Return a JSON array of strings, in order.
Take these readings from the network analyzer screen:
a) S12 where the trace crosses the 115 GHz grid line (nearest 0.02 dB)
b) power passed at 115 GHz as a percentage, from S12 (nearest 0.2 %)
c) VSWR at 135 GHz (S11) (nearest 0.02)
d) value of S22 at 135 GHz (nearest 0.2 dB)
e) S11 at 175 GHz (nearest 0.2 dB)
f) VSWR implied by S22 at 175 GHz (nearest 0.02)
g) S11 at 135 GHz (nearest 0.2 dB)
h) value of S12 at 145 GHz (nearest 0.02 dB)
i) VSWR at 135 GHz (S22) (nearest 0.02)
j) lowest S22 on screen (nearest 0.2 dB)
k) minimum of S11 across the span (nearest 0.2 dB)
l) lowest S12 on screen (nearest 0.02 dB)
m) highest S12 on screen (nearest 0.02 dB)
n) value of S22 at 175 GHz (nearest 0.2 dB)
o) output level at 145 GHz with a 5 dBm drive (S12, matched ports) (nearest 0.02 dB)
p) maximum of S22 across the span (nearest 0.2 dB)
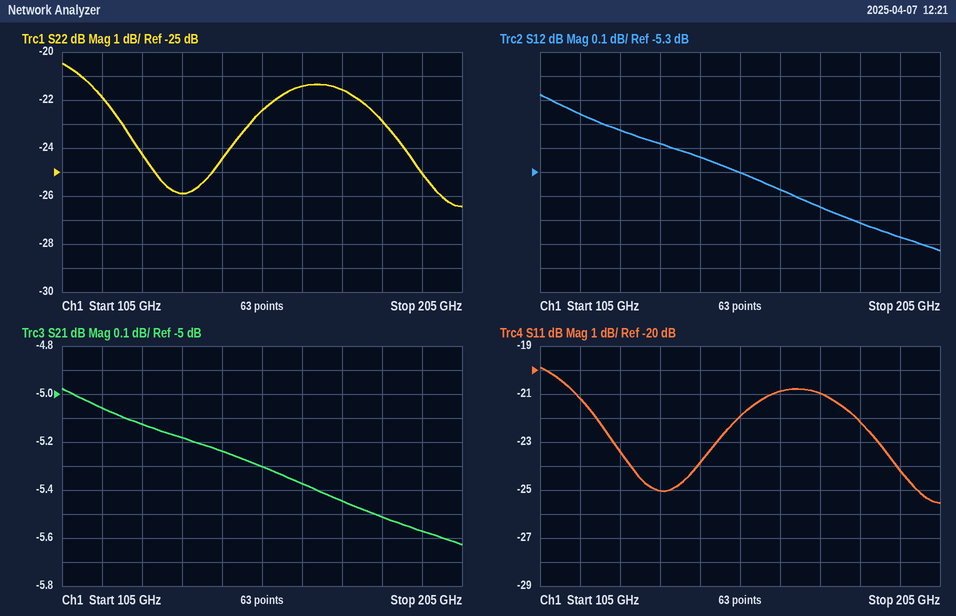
["-5.06 dB", "31.2 %", "1.12", "-25.8 dB", "-21.0 dB", "1.18", "-25.0 dB", "-5.24 dB", "1.10", "-26.4 dB", "-25.6 dB", "-5.62 dB", "-4.98 dB", "-21.6 dB", "-0.24 dBm", "-20.4 dB"]
